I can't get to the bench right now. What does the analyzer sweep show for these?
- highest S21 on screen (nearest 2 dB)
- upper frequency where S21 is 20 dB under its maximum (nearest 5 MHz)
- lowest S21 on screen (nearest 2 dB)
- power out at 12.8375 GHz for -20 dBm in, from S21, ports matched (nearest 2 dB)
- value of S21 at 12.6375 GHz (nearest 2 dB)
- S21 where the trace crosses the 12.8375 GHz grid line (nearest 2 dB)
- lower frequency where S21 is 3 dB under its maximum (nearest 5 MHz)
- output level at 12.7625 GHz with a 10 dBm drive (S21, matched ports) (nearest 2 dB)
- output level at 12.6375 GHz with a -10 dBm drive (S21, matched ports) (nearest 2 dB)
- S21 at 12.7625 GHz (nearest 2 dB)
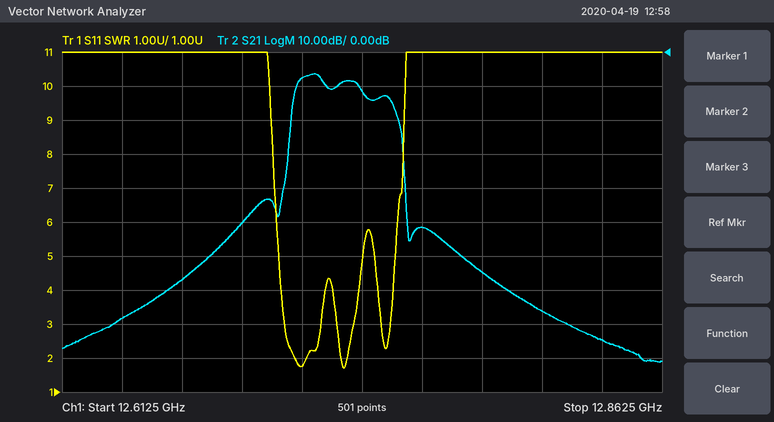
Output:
-6 dB
12.755 GHz
-92 dB
-104 dBm
-78 dB
-84 dB
12.710 GHz
-42 dBm
-88 dBm
-52 dB
